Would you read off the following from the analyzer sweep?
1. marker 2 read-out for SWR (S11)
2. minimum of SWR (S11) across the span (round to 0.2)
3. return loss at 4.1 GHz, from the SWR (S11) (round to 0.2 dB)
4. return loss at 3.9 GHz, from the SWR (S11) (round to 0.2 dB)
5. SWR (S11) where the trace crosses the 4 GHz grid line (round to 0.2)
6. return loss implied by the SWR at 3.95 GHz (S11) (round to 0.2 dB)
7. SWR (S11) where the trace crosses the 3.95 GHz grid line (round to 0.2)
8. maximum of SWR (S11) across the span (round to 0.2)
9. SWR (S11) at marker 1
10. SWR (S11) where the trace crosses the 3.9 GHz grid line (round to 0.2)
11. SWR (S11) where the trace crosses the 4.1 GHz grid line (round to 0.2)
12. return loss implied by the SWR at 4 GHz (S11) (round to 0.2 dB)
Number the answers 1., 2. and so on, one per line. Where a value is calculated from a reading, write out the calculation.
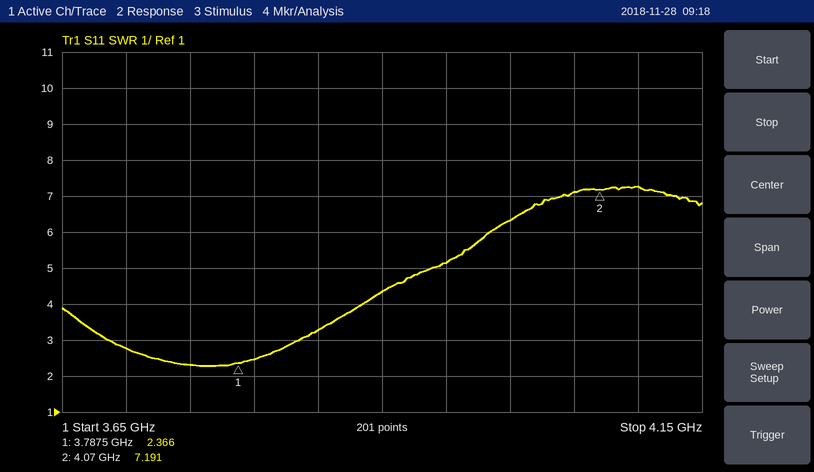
1. 7.191
2. 2.2
3. −20 log10((7.2 − 1)/(7.2 + 1)) ≈ 2.4 dB
4. −20 log10((4.4 − 1)/(4.4 + 1)) ≈ 4.0 dB
5. 6.4
6. −20 log10((5.2 − 1)/(5.2 + 1)) ≈ 3.4 dB
7. 5.2
8. 7.2
9. 2.366
10. 4.4
11. 7.2
12. −20 log10((6.4 − 1)/(6.4 + 1)) ≈ 2.74 dB, so 2.8 dB to the nearest 0.2 dB
